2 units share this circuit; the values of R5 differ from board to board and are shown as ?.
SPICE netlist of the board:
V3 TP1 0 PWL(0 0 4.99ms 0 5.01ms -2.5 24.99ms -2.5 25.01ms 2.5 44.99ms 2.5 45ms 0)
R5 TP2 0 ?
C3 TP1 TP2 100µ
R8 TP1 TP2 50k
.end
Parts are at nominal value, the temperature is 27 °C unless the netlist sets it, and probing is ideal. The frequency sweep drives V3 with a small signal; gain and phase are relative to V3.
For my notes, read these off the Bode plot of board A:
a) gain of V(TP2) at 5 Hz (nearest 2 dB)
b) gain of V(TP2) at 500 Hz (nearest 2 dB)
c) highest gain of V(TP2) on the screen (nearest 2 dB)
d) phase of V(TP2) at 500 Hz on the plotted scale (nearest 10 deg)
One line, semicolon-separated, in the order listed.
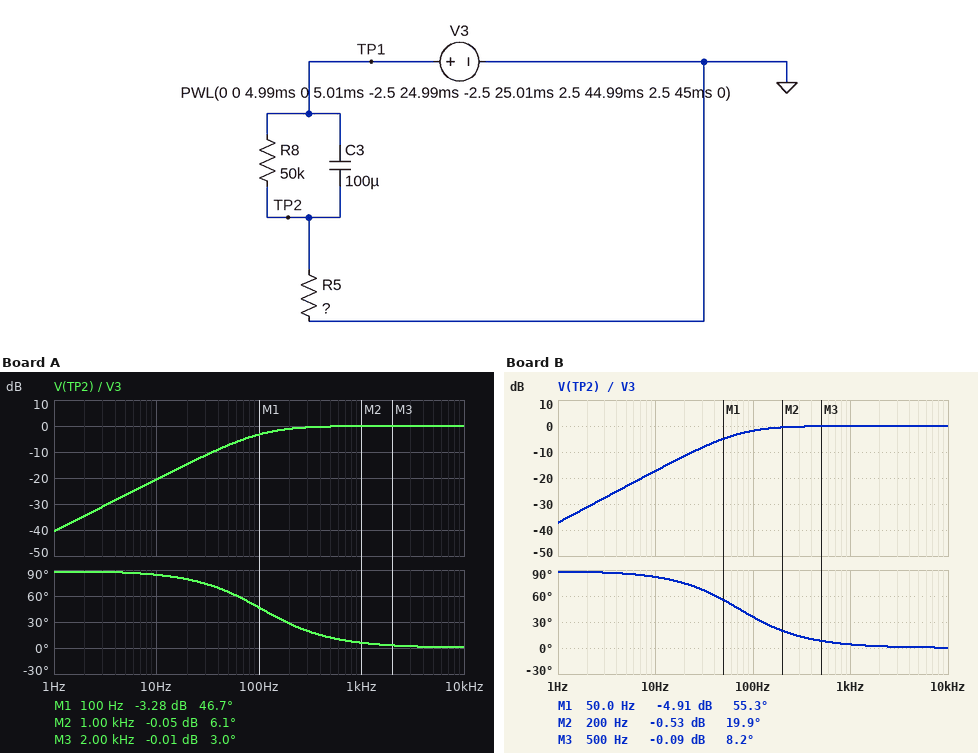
-26 dB; 0 dB; 0 dB; 10 deg
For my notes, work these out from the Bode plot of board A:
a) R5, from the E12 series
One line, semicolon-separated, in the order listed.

15 Ω
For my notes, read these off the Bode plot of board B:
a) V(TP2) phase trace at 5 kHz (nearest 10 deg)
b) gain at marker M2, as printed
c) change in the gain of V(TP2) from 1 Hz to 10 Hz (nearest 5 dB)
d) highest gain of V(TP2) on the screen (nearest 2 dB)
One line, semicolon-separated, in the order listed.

0 deg; -0.53 dB; 20 dB; 0 dB
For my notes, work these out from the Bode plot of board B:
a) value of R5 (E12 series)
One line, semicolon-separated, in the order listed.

22 Ω
